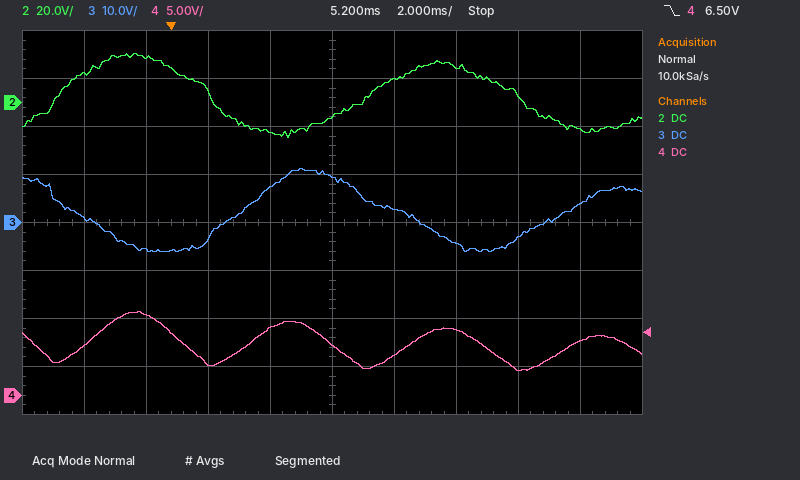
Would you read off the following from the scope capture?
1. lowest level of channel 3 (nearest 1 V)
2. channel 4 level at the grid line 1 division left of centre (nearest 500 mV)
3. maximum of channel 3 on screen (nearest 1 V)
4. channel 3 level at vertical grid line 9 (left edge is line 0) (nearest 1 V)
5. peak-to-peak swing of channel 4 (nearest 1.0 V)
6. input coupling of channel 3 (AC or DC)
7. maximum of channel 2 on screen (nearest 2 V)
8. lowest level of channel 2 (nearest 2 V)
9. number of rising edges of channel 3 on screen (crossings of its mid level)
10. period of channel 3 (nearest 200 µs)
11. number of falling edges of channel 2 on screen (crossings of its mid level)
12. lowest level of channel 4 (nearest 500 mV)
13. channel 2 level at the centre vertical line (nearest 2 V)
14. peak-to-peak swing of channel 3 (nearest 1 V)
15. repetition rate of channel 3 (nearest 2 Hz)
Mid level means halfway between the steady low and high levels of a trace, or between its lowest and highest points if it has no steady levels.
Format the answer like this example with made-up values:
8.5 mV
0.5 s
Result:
-6 V
7.0 V
11 V
4 V
6.0 V
DC
20 V
-14 V
2
10.6 ms
2
2.5 V
-6 V
17 V
94 Hz
